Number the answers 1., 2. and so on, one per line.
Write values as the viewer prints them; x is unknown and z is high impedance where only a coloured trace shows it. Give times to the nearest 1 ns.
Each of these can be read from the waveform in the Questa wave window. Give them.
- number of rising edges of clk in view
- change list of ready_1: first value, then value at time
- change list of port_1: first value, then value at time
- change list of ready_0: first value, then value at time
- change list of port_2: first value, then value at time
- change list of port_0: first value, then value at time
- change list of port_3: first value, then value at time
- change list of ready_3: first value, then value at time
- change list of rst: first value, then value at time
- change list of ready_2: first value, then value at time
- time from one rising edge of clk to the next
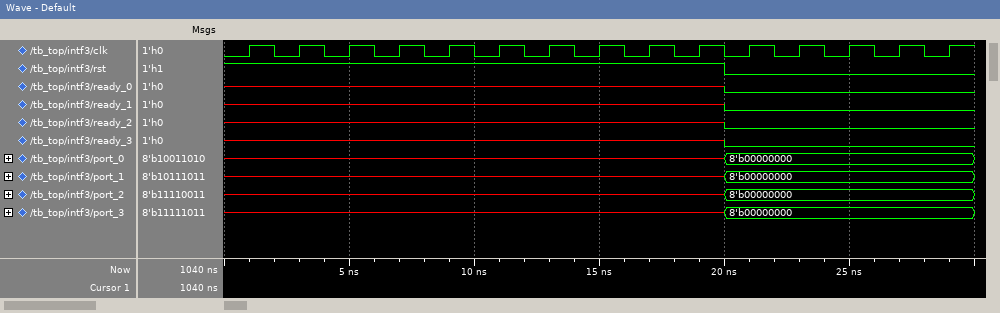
1. 15
2. x, 0 at 20 ns
3. x, 8'b00000000 at 20 ns
4. x, 0 at 20 ns
5. x, 8'b00000000 at 20 ns
6. x, 8'b00000000 at 20 ns
7. x, 8'b00000000 at 20 ns
8. x, 0 at 20 ns
9. 1, 0 at 20 ns
10. x, 0 at 20 ns
11. 2 ns
